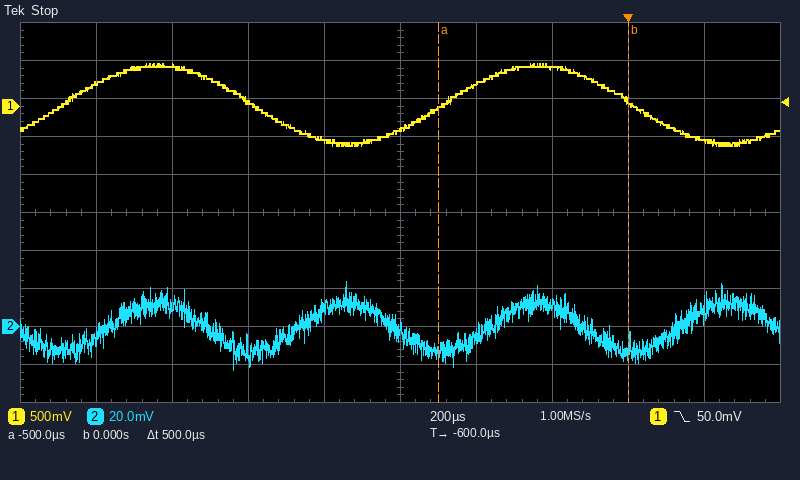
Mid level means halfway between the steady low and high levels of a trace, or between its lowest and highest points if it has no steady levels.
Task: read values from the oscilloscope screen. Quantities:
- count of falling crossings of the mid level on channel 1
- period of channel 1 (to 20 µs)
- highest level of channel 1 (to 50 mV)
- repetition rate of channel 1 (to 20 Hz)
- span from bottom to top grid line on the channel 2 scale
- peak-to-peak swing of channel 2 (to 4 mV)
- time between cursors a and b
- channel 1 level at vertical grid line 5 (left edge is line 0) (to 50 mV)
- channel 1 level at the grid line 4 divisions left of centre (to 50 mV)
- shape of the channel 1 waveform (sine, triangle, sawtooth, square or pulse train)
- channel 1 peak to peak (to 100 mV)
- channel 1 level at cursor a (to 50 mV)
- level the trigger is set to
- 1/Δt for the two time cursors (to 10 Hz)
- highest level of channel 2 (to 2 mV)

2
1.00 ms
550 mV
1.00 kHz
200 mV
48 mV
500 µs
-300 mV
300 mV
sine
1.10 V
0 mV
50.0 mV
2.00 kHz
24 mV
